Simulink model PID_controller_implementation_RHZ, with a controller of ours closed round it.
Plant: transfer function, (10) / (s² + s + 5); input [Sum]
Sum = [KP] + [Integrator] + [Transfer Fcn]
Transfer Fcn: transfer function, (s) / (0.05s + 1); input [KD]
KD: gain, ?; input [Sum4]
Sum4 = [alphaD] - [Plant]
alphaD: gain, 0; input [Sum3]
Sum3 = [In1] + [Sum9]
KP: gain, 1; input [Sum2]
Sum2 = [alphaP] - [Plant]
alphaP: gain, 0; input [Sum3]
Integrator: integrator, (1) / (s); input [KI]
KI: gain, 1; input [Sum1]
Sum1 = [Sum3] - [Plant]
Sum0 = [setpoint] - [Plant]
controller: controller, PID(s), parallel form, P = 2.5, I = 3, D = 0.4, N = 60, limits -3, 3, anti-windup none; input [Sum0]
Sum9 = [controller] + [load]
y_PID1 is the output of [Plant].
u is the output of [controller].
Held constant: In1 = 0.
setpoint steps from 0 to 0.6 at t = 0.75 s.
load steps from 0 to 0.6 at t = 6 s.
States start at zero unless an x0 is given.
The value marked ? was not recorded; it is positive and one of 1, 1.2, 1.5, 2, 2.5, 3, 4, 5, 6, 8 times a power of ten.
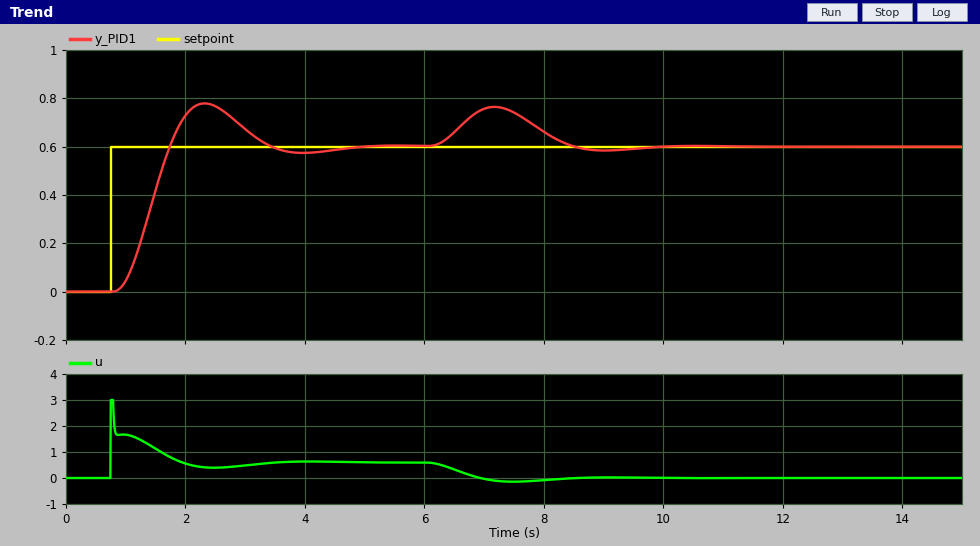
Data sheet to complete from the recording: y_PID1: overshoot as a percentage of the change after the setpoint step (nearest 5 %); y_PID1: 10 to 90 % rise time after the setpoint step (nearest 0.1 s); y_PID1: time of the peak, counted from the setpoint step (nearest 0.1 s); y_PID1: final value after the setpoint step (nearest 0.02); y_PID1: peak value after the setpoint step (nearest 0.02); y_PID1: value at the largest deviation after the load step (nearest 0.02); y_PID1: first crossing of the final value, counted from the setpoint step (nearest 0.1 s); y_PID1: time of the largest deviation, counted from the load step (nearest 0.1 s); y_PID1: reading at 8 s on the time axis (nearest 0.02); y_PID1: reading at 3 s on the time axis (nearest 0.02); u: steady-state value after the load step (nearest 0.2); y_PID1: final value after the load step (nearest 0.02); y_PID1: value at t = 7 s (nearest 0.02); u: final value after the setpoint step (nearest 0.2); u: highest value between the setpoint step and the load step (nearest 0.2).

30 %
0.6 s
1.6 s
0.60
0.78
0.76
1.0 s
1.2 s
0.66
0.68
0.0
0.60
0.76
0.6
3.0
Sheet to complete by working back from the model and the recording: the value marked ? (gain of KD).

0.5
